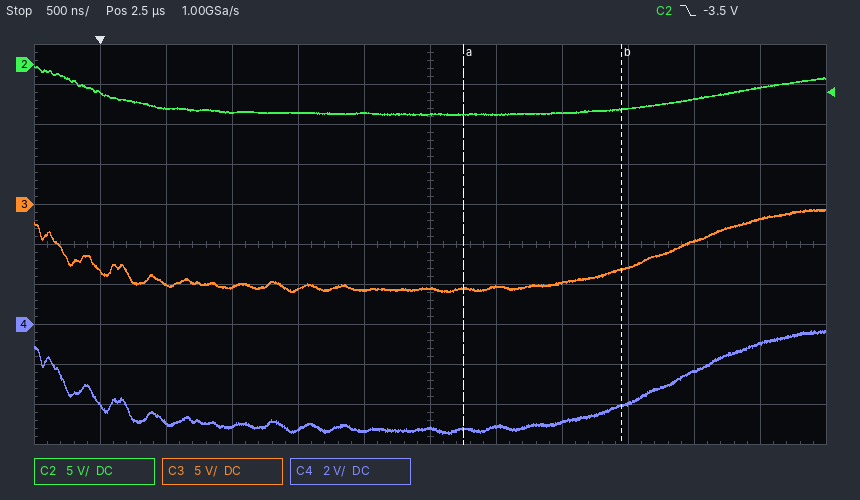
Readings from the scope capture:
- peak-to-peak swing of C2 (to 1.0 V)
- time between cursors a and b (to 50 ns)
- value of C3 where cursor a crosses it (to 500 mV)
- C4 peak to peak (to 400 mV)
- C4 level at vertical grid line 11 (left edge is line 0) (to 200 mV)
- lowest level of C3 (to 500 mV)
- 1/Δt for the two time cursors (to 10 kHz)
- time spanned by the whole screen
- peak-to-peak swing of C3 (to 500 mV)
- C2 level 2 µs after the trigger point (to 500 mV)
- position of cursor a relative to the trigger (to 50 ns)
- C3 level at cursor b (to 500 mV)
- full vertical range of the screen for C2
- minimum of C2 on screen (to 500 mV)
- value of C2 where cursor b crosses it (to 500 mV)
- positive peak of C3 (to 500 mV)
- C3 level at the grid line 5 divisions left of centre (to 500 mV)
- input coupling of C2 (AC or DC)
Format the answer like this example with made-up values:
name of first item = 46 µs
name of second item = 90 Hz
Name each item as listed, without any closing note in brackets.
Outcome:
peak-to-peak swing of C2 = 6.0 V
time between cursors a and b = 1.20 µs
value of C3 where cursor a crosses it = -10.5 V
C4 peak to peak = 5.2 V
C4 level at vertical grid line 11 (left edge is line 0) = -1.0 V
lowest level of C3 = -11.0 V
1/Δt for the two time cursors = 830 kHz
time spanned by the whole screen = 6 µs
peak-to-peak swing of C3 = 10.5 V
C2 level 2 µs after the trigger point = -6.0 V
position of cursor a relative to the trigger = +2.75 µs
C3 level at cursor b = -8.0 V
full vertical range of the screen for C2 = 50 V
minimum of C2 on screen = -6.5 V
value of C2 where cursor b crosses it = -5.5 V
positive peak of C3 = -500 mV
C3 level at the grid line 5 divisions left of centre = -8.5 V
input coupling of C2 = DC
